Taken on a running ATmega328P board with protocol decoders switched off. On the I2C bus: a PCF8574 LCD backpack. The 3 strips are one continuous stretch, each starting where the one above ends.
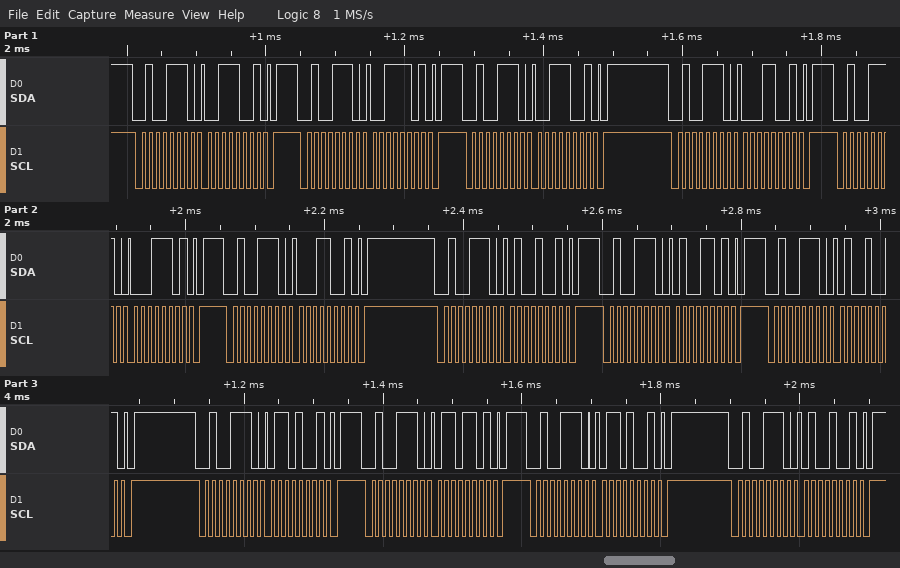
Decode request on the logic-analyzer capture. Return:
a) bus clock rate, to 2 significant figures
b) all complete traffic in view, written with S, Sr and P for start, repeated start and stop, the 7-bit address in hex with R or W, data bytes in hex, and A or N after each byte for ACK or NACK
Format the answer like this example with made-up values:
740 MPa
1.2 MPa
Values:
100 kHz
S 27W A 39 A P S 27W A 3D A P S 27W A 39 A P S 27W A 19 A P S 27W A 1D A P S 27W A 19 A P S 27W A 49 A P S 27W A 4D A P S 27W A 49 A P S 27W A 69 A P S 27W A 6D A P S 27W A 69 A P S 27W A 49 A P
